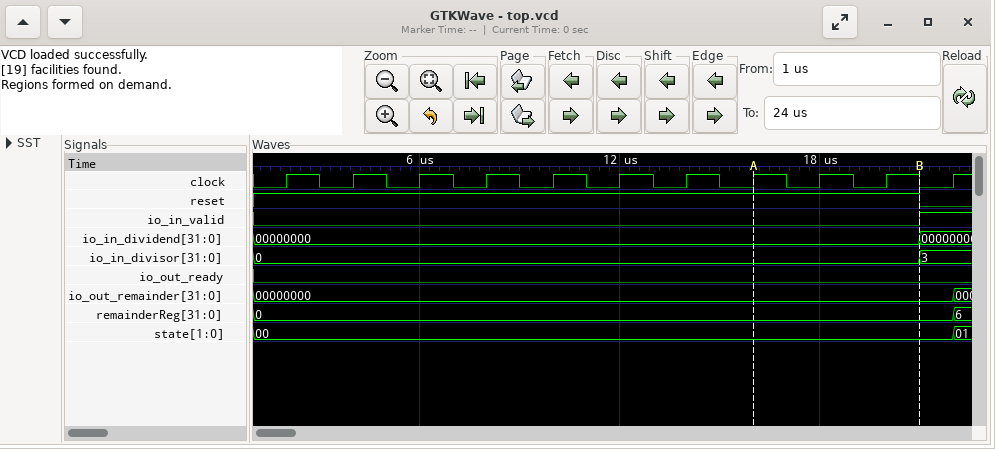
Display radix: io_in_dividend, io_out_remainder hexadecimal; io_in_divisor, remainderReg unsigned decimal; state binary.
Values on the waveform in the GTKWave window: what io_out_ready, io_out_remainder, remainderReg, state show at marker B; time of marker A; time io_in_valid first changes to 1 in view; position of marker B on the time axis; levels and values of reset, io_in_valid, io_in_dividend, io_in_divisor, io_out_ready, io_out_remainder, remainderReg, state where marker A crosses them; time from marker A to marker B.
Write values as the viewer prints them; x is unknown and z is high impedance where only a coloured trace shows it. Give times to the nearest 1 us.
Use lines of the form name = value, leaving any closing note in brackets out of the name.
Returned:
what io_out_ready, io_out_remainder, remainderReg, state show at marker B = io_out_ready=0, io_out_remainder=00000000, remainderReg=0, state=00
time of marker A = 16 us
time io_in_valid first changes to 1 in view = 21 us
position of marker B on the time axis = 21 us
levels and values of reset, io_in_valid, io_in_dividend, io_in_divisor, io_out_ready, io_out_remainder, remainderReg, state where marker A crosses them = reset=1, io_in_valid=0, io_in_dividend=00000000, io_in_divisor=0, io_out_ready=0, io_out_remainder=00000000, remainderReg=0, state=00
time from marker A to marker B = 5 us
